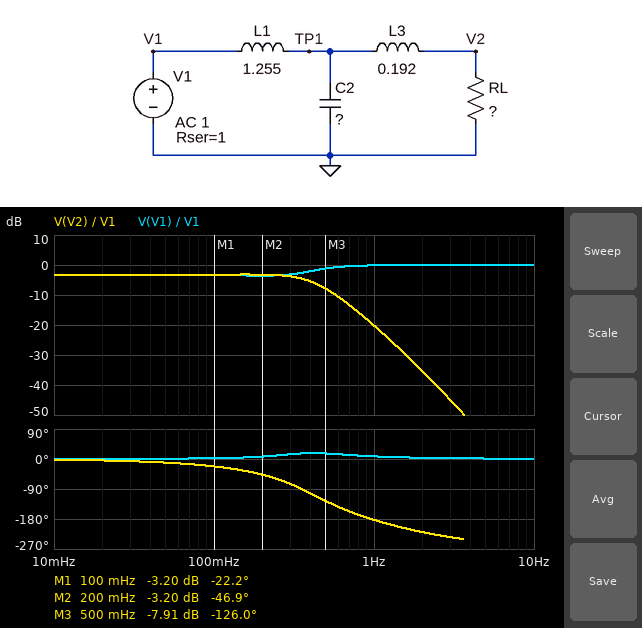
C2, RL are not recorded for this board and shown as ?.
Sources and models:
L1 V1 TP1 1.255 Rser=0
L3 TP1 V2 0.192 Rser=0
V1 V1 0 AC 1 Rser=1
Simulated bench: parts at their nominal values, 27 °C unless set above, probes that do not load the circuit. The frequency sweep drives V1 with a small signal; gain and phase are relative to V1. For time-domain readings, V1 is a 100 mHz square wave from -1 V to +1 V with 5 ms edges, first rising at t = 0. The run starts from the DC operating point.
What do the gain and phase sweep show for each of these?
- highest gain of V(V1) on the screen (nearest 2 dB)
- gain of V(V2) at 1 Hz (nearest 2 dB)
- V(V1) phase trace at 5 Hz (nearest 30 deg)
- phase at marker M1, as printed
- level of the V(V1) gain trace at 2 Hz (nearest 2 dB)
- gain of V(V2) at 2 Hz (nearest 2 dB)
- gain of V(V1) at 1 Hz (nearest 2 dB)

0 dB
-20 dB
0 deg
-22.2 deg
0 dB
-36 dB
0 dB
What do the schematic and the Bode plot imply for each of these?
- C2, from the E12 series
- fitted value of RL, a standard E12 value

220 mF
2.2 Ω
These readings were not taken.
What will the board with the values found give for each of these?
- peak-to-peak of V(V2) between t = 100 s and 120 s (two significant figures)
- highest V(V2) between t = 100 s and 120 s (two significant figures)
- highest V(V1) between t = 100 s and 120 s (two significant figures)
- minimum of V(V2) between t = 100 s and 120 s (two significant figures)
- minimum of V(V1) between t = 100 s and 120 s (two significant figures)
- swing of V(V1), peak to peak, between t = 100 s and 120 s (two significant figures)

1.6 V
780 mV
1.3 V
-780 mV
-1.3 V
2.6 V
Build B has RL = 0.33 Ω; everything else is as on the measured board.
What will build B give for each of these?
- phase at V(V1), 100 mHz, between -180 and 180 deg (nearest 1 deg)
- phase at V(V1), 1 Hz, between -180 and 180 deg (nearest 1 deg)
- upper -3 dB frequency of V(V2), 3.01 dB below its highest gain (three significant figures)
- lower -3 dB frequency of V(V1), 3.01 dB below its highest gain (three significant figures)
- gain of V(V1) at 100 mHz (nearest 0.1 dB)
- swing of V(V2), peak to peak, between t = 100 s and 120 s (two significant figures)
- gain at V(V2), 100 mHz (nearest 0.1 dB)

35 deg
9 deg
157 mHz
140 mHz
-4.5 dB
490 mV
-13.6 dB
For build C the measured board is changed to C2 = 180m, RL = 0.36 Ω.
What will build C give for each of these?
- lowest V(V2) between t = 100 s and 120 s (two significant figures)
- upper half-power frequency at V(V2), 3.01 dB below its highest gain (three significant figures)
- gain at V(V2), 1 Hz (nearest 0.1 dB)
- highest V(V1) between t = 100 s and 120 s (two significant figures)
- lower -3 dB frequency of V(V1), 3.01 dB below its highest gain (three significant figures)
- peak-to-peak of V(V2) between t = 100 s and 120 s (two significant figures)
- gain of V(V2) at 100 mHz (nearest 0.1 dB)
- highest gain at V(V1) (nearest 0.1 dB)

-260 mV
159 mHz
-19.6 dB
1.7 V
142 mHz
520 mV
-13.0 dB
0 dB
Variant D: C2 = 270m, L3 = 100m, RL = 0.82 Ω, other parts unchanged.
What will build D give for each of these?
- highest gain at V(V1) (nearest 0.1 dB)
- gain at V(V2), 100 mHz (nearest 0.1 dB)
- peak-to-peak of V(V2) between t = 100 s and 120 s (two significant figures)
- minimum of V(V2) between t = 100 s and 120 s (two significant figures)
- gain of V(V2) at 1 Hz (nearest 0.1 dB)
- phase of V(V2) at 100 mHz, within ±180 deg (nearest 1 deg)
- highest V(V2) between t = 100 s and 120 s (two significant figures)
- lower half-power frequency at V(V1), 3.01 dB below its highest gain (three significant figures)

0 dB
-7.6 dB
900 mV
-450 mV
-22.0 dB
-30 deg
450 mV
191 mHz
